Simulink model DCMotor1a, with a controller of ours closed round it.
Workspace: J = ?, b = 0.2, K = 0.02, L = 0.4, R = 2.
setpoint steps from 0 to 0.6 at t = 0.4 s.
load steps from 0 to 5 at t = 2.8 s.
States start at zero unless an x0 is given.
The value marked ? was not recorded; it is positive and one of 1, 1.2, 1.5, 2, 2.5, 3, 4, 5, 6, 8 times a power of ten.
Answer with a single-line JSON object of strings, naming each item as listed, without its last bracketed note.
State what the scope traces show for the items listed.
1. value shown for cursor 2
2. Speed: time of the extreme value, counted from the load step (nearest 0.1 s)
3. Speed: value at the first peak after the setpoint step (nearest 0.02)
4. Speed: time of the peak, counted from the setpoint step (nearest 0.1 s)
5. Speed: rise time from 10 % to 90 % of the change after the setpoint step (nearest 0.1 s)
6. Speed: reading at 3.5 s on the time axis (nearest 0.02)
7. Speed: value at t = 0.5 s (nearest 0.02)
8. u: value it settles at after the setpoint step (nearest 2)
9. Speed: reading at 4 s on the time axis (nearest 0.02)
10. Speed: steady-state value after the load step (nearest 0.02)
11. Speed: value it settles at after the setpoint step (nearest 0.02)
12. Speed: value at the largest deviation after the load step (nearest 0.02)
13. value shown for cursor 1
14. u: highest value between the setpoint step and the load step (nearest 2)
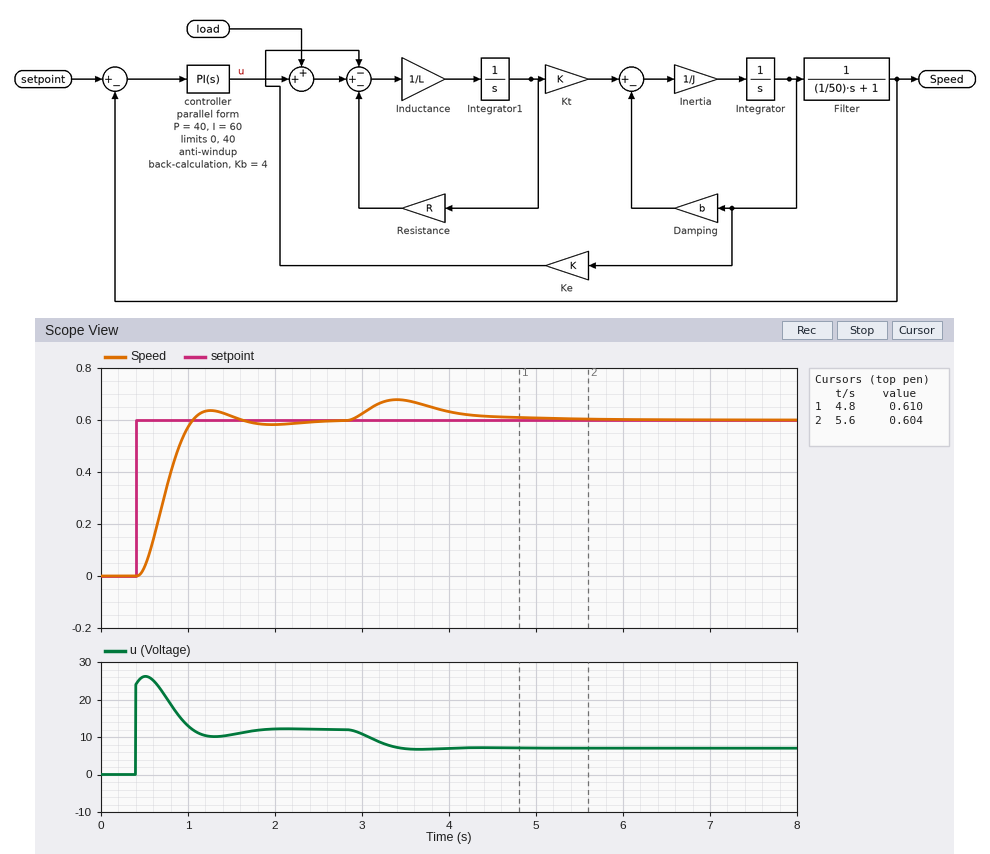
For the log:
{"value shown for cursor 2": "0.604", "Speed: time of the extreme value, counted from the load step": "0.6 s", "Speed: value at the first peak after the setpoint step": "0.64", "Speed: time of the peak, counted from the setpoint step": "0.9 s", "Speed: rise time from 10 % to 90 % of the change after the setpoint step": "0.4 s", "Speed: reading at 3.5 s on the time axis": "0.68", "Speed: value at t = 0.5 s": "0.04", "u: value it settles at after the setpoint step": "12", "Speed: reading at 4 s on the time axis": "0.64", "Speed: steady-state value after the load step": "0.60", "Speed: value it settles at after the setpoint step": "0.60", "Speed: value at the largest deviation after the load step": "0.68", "value shown for cursor 1": "0.610", "u: highest value between the setpoint step and the load step": "26"}
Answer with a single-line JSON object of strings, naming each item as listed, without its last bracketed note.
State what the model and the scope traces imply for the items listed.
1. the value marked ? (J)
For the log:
{"the value marked ?": "0.1"}
